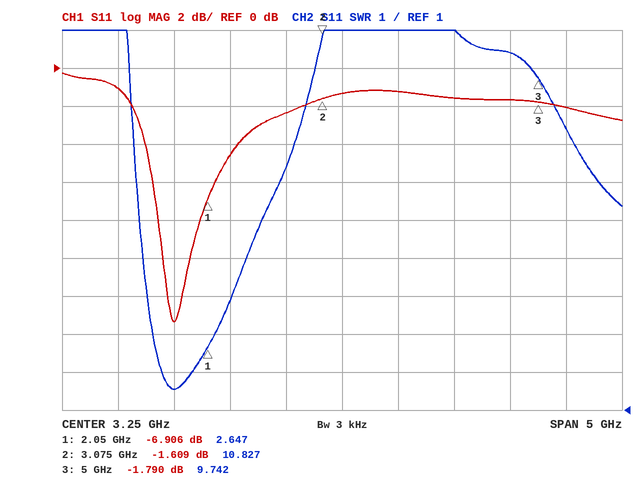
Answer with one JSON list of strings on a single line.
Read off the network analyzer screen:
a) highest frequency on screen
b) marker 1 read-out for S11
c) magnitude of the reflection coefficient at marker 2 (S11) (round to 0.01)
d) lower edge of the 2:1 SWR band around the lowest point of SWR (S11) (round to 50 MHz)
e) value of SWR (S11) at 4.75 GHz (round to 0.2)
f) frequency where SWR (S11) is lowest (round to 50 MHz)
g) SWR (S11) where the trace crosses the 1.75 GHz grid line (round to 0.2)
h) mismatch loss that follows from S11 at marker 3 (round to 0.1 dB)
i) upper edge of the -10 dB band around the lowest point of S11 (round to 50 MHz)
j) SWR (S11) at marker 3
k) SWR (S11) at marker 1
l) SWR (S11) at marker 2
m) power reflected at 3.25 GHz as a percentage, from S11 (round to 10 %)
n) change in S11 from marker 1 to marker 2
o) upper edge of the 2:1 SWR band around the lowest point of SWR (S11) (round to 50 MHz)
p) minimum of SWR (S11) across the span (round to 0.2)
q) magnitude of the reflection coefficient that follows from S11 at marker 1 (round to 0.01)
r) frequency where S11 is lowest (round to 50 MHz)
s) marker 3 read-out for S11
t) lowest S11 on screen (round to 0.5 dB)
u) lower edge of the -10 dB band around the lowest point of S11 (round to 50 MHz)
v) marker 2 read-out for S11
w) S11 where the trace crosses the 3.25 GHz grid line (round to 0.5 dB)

["5.75 GHz", "-6.906 dB", "0.83", "1.65 GHz", "10.4", "1.75 GHz", "1.6", "4.7 dB", "1.90 GHz", "9.742", "2.647", "10.827", "70 %", "5.297 dB", "1.90 GHz", "1.6", "0.45", "1.75 GHz", "-1.790 dB", "-13.5 dB", "1.65 GHz", "-1.609 dB", "-1.5 dB"]
